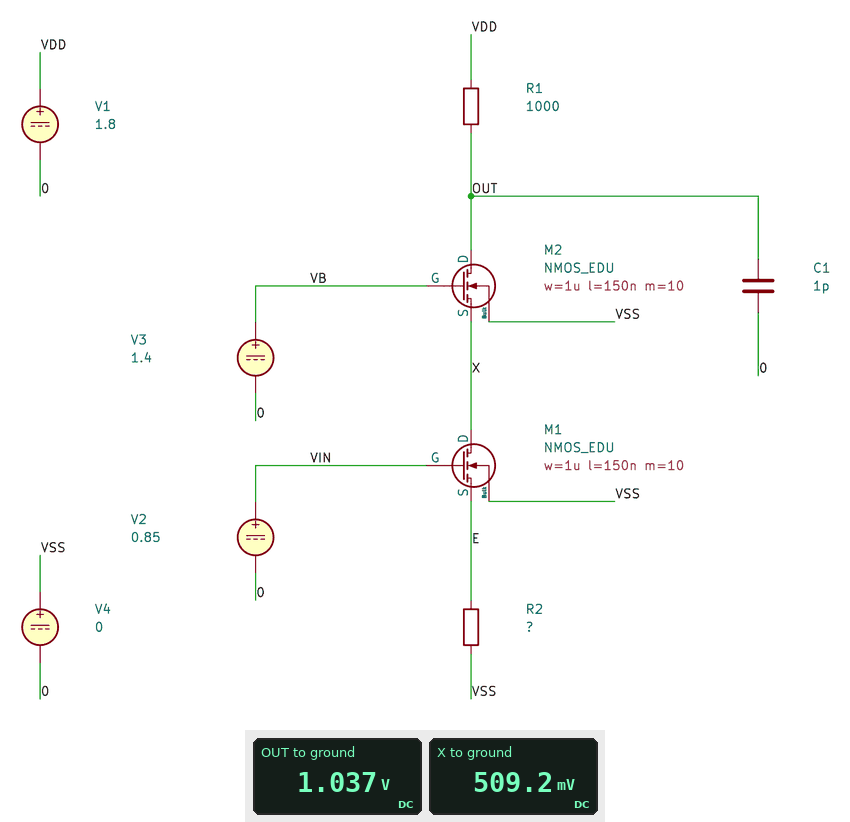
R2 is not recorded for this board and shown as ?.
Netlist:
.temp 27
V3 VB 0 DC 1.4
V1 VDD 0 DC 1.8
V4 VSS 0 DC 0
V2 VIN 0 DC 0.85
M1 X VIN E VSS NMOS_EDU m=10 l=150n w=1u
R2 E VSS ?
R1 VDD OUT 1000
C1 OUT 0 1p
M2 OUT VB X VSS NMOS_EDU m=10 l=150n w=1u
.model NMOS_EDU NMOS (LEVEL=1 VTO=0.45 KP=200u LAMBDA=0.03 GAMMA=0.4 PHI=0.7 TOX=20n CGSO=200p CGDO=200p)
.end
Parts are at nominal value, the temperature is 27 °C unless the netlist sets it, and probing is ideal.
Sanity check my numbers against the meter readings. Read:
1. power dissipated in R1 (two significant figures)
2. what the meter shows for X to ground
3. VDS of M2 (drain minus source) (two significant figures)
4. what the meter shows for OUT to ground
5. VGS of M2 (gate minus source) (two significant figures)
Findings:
580 µW
509.2 mV
530 mV
1.037 V
890 mV
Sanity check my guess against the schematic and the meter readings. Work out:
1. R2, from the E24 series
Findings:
68 Ω
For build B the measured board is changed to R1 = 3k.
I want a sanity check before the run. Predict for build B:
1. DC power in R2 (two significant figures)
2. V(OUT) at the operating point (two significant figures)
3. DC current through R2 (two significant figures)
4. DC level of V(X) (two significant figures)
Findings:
19 µW
230 mV
520 µA
170 mV
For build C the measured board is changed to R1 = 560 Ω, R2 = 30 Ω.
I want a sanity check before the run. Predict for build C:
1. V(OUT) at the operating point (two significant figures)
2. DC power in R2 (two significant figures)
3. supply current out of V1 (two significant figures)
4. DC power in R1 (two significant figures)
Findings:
1.3 V
25 µW
910 µA
460 µW
